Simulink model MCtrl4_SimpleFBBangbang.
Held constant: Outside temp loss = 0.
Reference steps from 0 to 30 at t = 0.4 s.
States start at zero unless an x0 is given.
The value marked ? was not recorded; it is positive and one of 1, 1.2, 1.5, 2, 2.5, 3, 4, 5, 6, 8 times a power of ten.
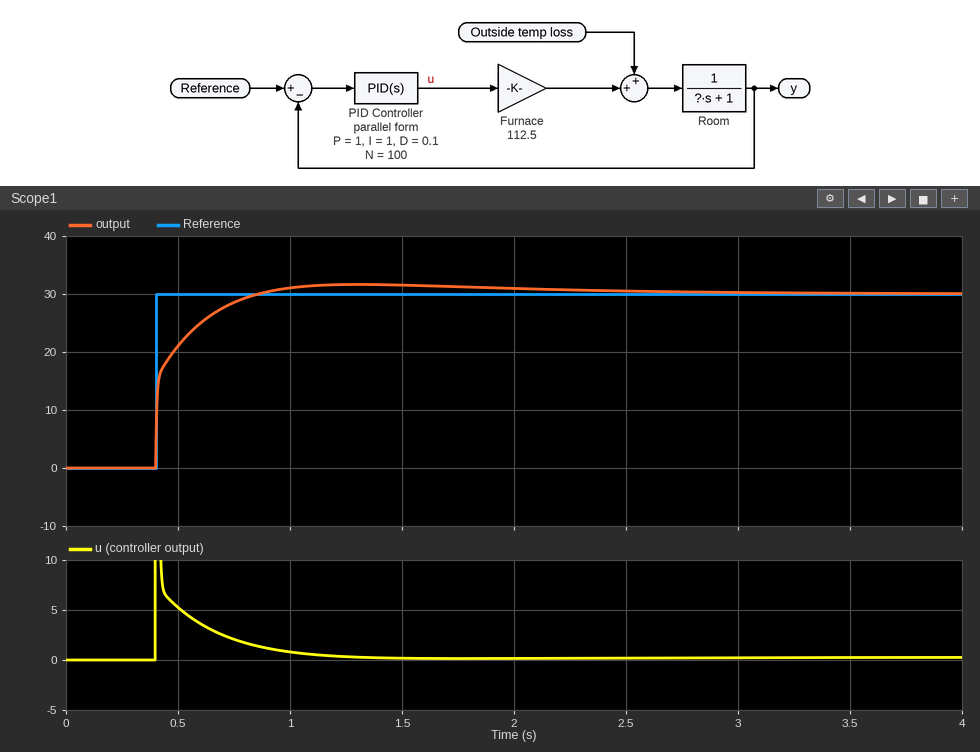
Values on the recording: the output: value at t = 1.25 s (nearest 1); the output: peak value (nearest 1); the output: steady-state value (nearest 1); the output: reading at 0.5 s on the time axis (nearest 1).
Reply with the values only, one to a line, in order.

32
32
30
21
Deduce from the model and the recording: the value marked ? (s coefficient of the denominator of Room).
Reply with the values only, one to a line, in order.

12
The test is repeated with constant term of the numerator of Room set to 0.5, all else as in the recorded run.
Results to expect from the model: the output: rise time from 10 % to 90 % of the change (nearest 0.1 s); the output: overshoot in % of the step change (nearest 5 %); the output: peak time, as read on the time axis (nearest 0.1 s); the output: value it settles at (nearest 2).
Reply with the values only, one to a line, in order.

0.4 s
10 %
1.6 s
30
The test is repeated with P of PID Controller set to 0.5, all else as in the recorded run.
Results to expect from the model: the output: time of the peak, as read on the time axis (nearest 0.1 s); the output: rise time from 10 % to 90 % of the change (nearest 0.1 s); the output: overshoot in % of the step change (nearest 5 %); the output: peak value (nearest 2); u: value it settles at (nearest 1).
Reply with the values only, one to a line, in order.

1.5 s
0.4 s
15 %
34
0
